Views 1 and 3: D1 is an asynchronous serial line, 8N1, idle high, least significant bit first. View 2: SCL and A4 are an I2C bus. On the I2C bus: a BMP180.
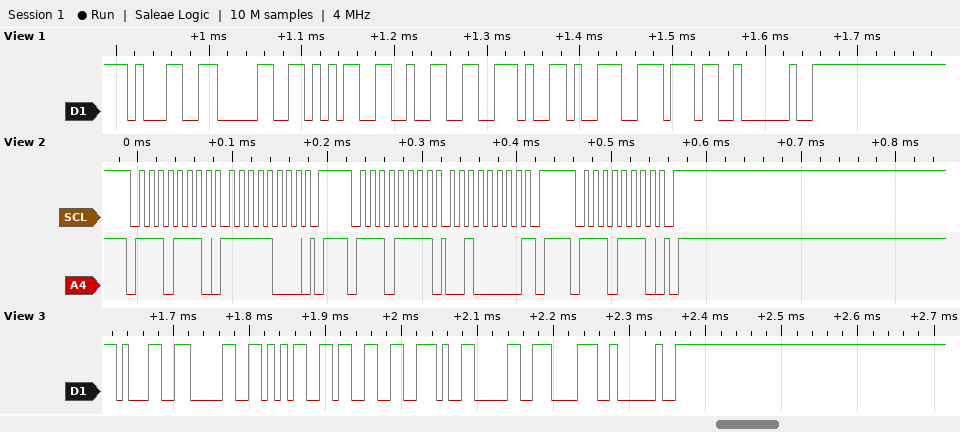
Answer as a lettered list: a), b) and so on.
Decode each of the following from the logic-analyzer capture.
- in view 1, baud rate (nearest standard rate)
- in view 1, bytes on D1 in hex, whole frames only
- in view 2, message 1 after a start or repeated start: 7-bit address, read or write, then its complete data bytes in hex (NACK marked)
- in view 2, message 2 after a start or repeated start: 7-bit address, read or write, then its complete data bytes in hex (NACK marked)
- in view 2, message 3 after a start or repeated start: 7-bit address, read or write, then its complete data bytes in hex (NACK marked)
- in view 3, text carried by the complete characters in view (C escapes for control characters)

a) 115200 baud
b) 0x31 0x30 0x35 0x32 0x2E 0x39 0x37 0x20
c) 0x77 write: F8
d) 0x77 read: 20 NACK
e) 0x77 write
f) "1053.08 "
